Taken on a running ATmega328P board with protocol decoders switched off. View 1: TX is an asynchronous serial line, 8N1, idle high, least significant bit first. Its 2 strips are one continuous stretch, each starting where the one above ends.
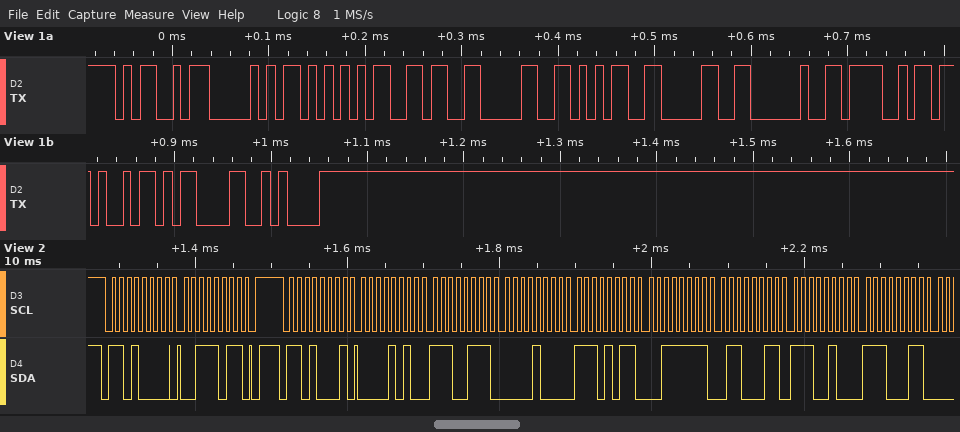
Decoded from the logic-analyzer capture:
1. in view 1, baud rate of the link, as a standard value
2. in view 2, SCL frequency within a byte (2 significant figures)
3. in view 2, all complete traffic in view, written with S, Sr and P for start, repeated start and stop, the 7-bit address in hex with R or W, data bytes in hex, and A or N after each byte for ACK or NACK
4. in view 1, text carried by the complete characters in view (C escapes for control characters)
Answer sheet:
115200 baud
100 kHz
S 68W A 3B A P S 68R A 0A A E7 A 08 A EB A 3F A 63 A E4 A E3 A
"MPU6050 OK\r\n"
